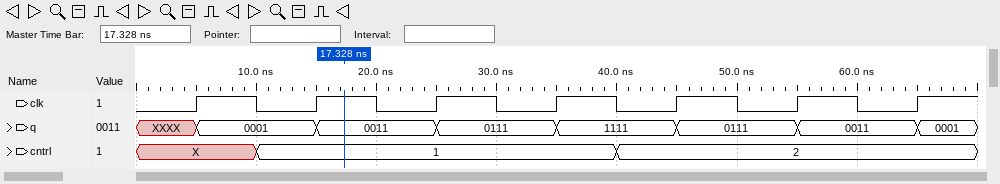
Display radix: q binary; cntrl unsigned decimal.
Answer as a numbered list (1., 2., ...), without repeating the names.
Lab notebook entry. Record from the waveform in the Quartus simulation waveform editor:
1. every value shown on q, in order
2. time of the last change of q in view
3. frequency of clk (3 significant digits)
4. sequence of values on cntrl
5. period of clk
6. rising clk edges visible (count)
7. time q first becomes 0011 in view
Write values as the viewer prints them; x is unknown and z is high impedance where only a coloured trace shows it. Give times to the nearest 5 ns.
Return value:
1. XXXX, 0001, 0011, 0111, 1111, 0111, 0011, 0001
2. 65 ns
3. 100 MHz
4. X, 1, 2
5. 10 ns
6. 7
7. 15 ns
